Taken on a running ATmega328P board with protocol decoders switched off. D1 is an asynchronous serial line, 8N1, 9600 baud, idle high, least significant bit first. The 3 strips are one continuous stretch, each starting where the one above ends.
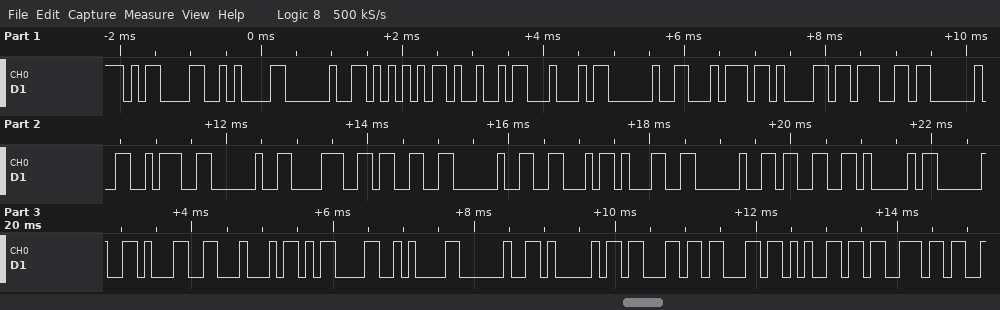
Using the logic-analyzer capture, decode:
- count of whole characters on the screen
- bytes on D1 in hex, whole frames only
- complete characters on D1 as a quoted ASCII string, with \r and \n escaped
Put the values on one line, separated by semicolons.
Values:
32; 0D 0A 20 55 49 44 20 74 61 67 20 3A 20 38 33 20 46 31 20 33 41 20 31 44 0D 0A 20 41 63 63 65 73; "\r\n UID tag : 83 F1 3A 1D\r\n Acces"
